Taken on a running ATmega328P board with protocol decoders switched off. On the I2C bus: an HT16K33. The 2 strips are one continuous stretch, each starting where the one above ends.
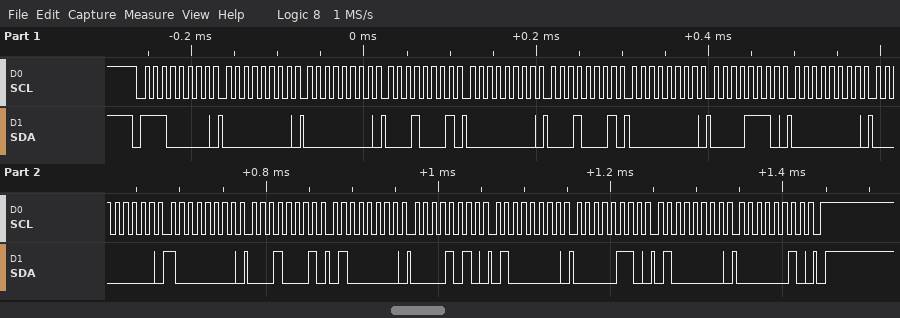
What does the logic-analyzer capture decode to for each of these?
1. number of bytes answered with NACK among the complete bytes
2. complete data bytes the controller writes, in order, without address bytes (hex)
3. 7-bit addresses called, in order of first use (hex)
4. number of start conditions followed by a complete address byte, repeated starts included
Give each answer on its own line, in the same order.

0
00 00 11 00 11 00 0E 00 00 80 11 40 0A 40 06 40 02
0x70
1
